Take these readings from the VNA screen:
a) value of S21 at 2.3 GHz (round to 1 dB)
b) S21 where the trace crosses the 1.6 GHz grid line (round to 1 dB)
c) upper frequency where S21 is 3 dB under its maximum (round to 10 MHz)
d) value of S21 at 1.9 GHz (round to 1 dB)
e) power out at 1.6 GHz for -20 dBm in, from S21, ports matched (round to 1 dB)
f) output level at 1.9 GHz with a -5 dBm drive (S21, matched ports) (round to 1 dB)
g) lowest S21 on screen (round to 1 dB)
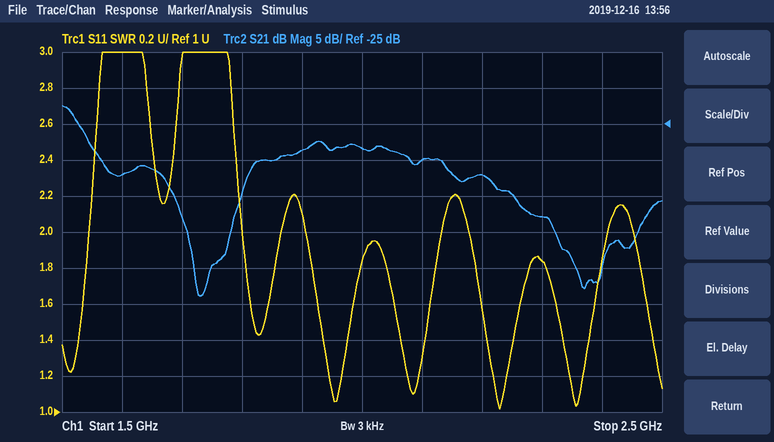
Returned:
-38 dB
-32 dB
1.53 GHz
-29 dB
-52 dBm
-34 dBm
-49 dB
